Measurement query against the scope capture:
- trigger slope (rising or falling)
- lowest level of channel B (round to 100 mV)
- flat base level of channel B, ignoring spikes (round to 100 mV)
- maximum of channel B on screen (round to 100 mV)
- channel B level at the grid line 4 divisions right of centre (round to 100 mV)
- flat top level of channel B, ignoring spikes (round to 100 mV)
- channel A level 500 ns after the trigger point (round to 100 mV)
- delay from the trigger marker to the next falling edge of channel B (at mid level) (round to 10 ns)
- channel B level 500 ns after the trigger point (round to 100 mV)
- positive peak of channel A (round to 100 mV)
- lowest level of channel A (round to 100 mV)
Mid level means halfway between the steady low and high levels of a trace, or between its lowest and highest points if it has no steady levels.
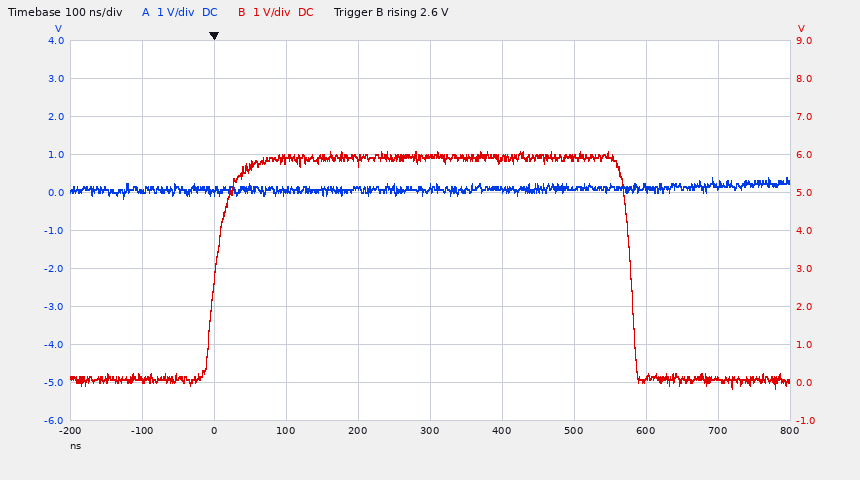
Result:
rising
-200 mV
100 mV
6.1 V
100 mV
5.9 V
100 mV
580 ns
5.9 V
400 mV
-200 mV
